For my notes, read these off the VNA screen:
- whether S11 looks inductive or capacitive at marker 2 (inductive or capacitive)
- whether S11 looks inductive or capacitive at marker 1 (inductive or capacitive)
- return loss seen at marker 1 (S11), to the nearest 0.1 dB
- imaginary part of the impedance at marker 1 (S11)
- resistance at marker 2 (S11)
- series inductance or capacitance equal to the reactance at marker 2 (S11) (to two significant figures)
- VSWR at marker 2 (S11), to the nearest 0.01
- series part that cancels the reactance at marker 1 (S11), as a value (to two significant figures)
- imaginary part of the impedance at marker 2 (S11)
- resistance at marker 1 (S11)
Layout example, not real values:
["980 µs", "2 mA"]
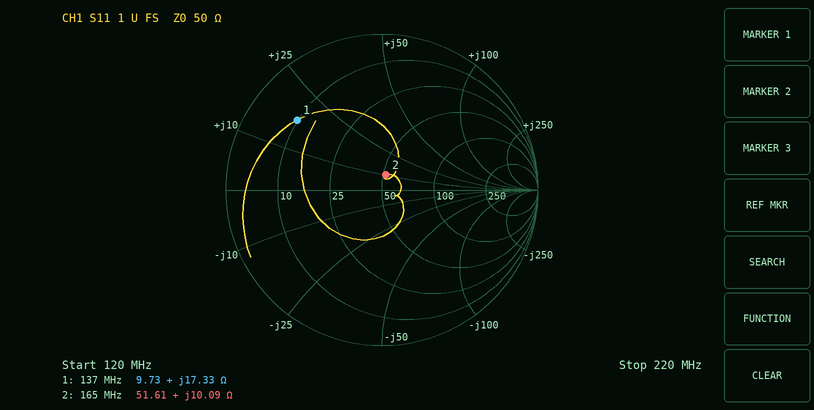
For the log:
["inductive", "inductive", "3.0 dB", "+17.33 Ω", "51.61 Ω", "9.7 nH", "1.22", "67 pF", "+10.09 Ω", "9.73 Ω"]
